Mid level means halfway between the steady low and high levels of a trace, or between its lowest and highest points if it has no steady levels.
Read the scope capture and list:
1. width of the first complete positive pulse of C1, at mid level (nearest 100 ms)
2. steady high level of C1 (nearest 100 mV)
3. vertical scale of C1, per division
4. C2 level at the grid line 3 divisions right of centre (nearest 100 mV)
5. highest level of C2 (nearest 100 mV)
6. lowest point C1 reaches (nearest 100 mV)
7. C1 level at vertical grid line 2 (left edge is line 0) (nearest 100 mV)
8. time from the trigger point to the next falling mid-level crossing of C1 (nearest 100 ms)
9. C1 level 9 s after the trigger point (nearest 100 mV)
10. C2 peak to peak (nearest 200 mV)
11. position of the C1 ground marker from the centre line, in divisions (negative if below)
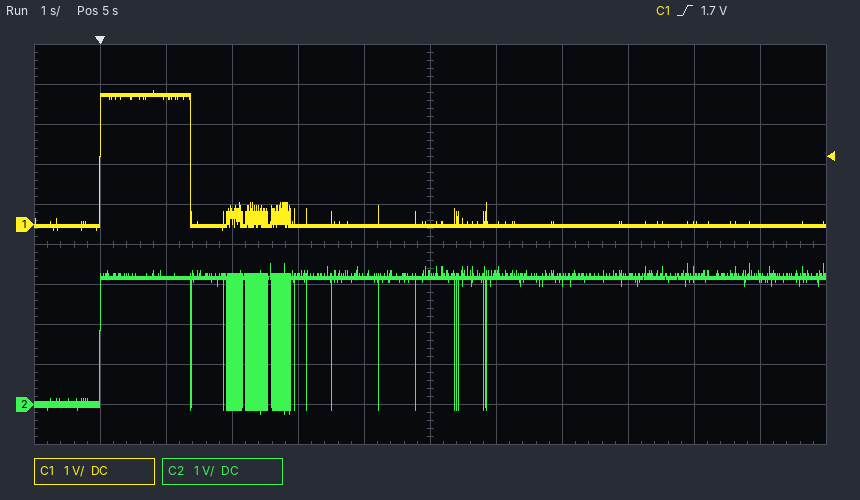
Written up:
1.4 s
3.2 V
1 V
3.2 V
3.5 V
-200 mV
3.2 V
1.4 s
0.0 V
3.8 V
+0.5 div
